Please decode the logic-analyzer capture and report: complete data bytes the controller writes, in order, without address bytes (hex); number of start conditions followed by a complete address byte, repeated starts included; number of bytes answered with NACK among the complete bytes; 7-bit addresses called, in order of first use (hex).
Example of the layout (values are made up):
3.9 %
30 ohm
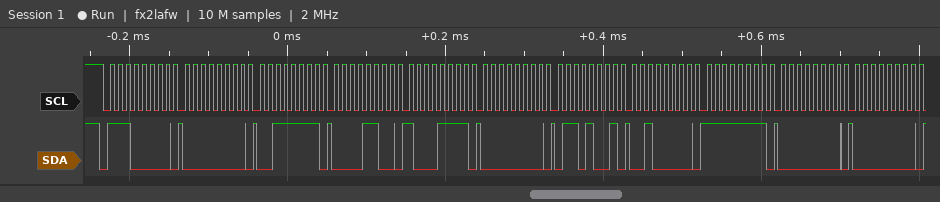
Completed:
00 3F 0C 8F 00 69 20 FF 00 00
1
0
0x70
